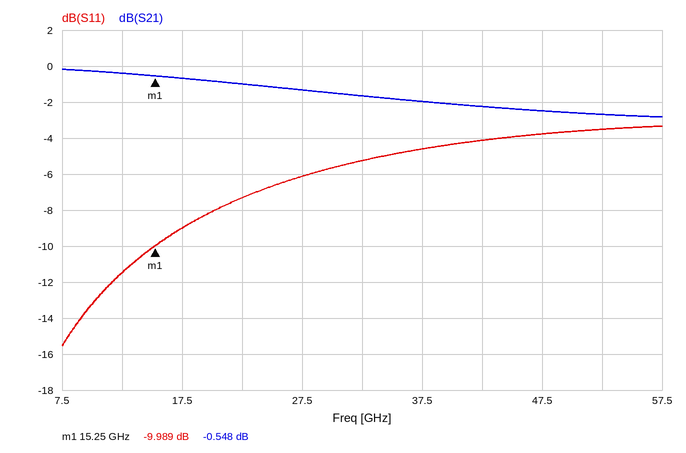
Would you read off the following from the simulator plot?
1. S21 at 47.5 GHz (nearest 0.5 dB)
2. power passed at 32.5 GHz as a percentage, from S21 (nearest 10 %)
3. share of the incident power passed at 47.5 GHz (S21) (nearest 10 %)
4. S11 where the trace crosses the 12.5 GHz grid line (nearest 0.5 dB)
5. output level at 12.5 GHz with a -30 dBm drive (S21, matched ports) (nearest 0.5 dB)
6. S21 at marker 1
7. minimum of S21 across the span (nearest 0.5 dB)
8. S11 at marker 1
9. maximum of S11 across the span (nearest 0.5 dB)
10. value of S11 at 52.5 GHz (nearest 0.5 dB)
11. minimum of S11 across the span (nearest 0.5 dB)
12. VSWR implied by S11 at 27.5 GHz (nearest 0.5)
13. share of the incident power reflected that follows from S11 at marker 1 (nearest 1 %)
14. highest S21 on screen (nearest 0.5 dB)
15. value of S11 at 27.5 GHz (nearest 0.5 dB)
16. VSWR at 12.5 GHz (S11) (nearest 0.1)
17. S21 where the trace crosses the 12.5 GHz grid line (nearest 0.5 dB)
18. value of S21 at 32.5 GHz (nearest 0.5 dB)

-2.5 dB
70 %
60 %
-11.5 dB
-30.5 dBm
-0.548 dB
-3.0 dB
-9.989 dB
-3.5 dB
-3.5 dB
-15.5 dB
3.0
10 %
0.0 dB
-6.0 dB
1.7
-0.5 dB
-1.5 dB
